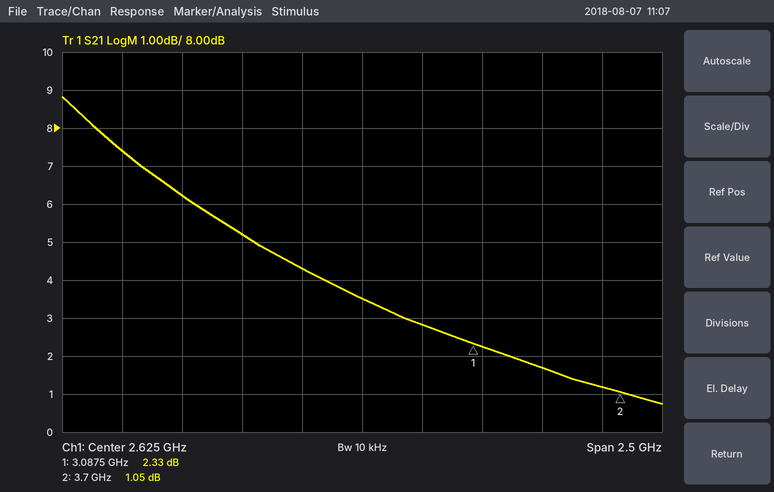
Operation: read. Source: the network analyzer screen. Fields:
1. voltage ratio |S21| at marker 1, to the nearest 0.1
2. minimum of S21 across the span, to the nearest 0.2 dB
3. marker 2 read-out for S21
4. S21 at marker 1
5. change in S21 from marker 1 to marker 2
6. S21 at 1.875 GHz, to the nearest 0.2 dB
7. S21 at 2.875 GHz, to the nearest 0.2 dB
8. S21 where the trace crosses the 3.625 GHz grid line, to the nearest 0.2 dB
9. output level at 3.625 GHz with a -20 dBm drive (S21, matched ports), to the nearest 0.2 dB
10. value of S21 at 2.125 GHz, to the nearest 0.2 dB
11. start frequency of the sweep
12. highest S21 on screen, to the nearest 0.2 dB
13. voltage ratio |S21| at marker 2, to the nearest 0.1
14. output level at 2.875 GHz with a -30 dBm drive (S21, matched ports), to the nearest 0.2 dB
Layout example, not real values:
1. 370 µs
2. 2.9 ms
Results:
1. 1.3
2. 0.8 dB
3. 1.05 dB
4. 2.33 dB
5. -1.28 dB
6. 6.2 dB
7. 2.8 dB
8. 1.2 dB
9. -18.8 dBm
10. 5.2 dB
11. 1.375 GHz
12. 8.8 dB
13. 1.1
14. -27.2 dBm
